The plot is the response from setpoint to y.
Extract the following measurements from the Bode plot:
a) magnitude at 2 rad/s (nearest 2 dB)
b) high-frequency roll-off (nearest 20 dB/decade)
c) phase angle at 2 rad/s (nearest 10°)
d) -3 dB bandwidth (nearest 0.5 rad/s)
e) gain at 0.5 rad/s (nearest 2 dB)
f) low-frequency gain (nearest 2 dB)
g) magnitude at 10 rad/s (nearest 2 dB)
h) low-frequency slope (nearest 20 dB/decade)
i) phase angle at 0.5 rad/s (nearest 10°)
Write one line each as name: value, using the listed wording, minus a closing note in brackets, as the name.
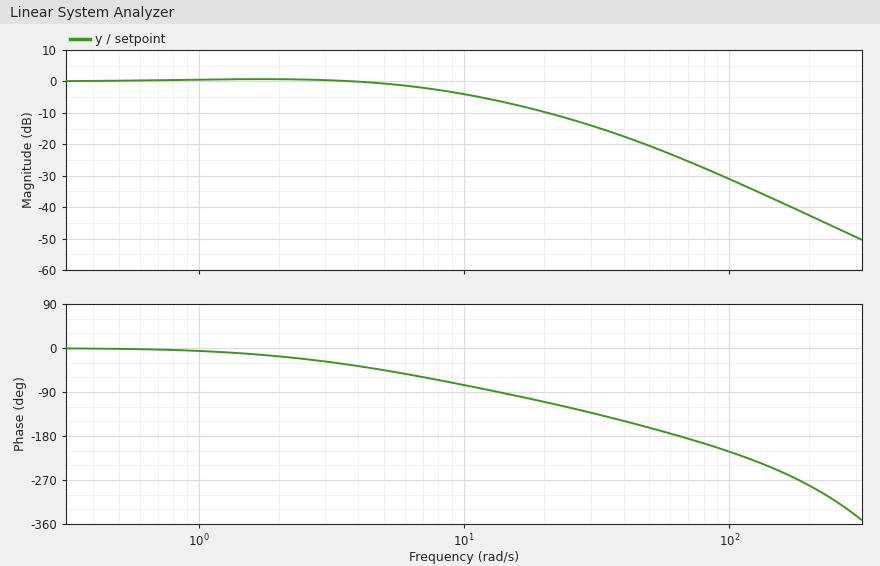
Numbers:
magnitude at 2 rad/s: 0 dB
high-frequency roll-off: -40 dB/decade
phase angle at 2 rad/s: -20°
-3 dB bandwidth: 8.0 rad/s
gain at 0.5 rad/s: 0 dB
low-frequency gain: 0 dB
magnitude at 10 rad/s: -4 dB
low-frequency slope: 0 dB/decade
phase angle at 0.5 rad/s: 0°
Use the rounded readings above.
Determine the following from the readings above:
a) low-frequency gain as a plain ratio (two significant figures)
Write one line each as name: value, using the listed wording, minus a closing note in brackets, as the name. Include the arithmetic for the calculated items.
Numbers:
low-frequency gain as a plain ratio: 10^(0 / 20) = 1.0
